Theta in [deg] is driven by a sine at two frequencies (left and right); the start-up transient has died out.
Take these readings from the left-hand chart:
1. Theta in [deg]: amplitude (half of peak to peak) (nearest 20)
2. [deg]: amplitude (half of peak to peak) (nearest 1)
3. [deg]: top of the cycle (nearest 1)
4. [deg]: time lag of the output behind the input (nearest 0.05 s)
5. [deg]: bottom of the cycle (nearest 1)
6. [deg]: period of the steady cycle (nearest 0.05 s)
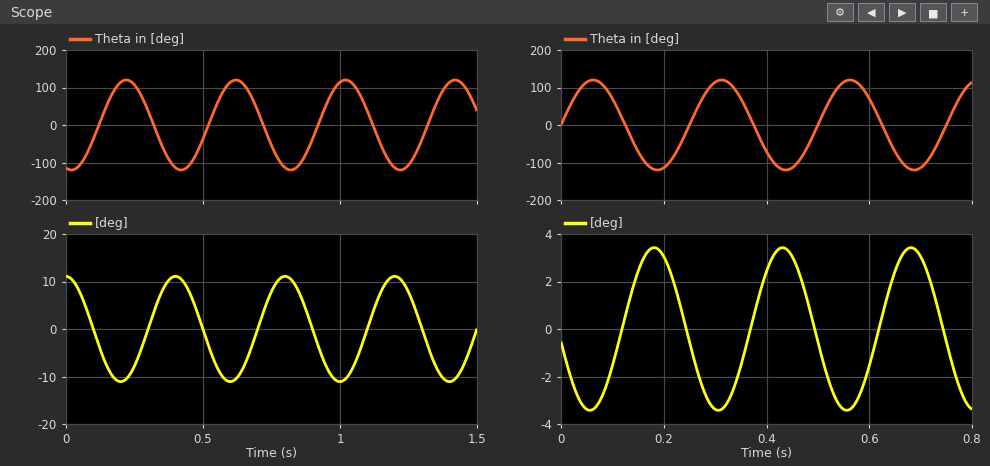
120
11
11
0.20 s
-11
0.40 s
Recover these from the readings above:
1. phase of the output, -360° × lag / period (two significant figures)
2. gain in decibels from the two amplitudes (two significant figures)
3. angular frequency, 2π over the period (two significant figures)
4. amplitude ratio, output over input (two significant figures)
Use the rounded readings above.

-180°
-21 dB
16 rad/s
0.092
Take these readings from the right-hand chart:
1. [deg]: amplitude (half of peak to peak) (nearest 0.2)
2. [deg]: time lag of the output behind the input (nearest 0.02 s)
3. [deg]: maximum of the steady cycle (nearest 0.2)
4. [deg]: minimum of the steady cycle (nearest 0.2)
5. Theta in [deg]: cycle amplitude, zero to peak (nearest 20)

3.4
0.12 s
3.4
-3.4
120
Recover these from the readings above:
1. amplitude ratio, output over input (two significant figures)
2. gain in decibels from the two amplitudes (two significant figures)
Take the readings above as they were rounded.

0.028
-31 dB
